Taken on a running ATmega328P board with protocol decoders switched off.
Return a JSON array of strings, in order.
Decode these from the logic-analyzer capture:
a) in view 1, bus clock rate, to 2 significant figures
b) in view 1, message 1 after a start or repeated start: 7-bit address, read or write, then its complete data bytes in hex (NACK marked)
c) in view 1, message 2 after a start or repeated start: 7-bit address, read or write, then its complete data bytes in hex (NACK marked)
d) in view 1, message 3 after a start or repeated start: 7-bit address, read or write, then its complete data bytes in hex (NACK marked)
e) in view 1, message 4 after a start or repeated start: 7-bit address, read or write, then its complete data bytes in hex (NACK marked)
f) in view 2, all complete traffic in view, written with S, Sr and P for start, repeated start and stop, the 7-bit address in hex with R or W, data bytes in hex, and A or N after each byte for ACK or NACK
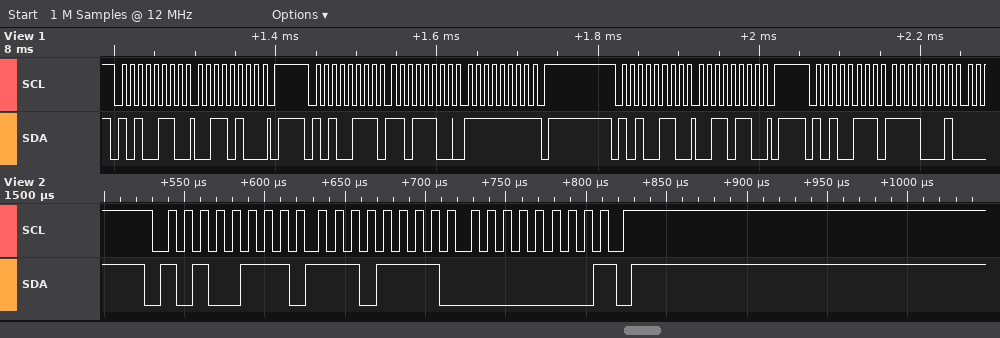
["100 kHz", "0x53 write: 34", "0x53 read: DC FF NACK", "0x53 write: 36", "0x53 read: F1", "S 53R A EF A 00 N P"]
